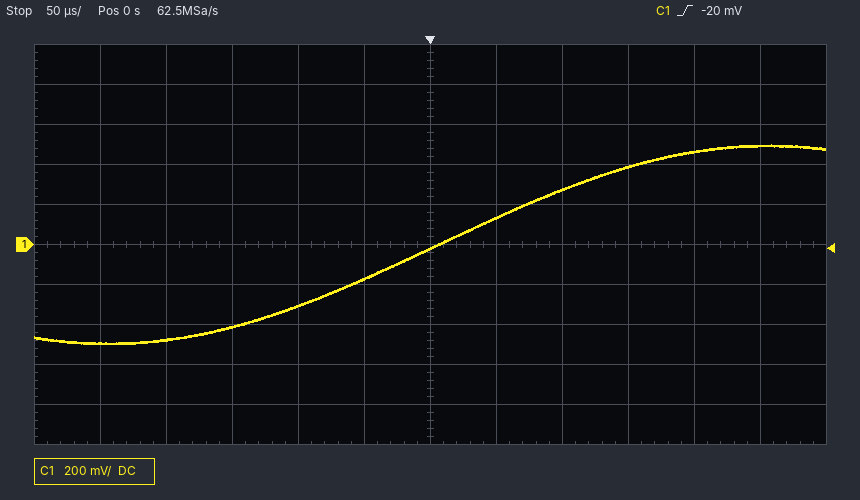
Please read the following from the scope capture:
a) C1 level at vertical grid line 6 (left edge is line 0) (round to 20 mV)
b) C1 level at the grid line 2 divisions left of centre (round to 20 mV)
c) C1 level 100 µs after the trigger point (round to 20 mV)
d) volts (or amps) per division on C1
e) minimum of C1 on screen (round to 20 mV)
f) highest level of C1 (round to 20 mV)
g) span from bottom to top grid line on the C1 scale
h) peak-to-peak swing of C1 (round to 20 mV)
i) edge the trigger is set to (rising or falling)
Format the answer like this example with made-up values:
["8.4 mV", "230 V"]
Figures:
["-20 mV", "-300 mV", "280 mV", "200 mV", "-500 mV", "500 mV", "2 V", "1.00 V", "rising"]
